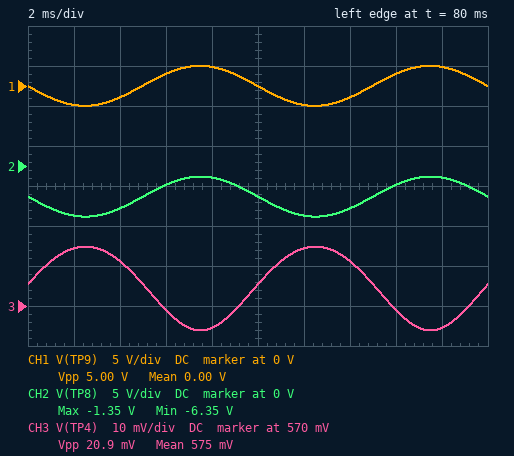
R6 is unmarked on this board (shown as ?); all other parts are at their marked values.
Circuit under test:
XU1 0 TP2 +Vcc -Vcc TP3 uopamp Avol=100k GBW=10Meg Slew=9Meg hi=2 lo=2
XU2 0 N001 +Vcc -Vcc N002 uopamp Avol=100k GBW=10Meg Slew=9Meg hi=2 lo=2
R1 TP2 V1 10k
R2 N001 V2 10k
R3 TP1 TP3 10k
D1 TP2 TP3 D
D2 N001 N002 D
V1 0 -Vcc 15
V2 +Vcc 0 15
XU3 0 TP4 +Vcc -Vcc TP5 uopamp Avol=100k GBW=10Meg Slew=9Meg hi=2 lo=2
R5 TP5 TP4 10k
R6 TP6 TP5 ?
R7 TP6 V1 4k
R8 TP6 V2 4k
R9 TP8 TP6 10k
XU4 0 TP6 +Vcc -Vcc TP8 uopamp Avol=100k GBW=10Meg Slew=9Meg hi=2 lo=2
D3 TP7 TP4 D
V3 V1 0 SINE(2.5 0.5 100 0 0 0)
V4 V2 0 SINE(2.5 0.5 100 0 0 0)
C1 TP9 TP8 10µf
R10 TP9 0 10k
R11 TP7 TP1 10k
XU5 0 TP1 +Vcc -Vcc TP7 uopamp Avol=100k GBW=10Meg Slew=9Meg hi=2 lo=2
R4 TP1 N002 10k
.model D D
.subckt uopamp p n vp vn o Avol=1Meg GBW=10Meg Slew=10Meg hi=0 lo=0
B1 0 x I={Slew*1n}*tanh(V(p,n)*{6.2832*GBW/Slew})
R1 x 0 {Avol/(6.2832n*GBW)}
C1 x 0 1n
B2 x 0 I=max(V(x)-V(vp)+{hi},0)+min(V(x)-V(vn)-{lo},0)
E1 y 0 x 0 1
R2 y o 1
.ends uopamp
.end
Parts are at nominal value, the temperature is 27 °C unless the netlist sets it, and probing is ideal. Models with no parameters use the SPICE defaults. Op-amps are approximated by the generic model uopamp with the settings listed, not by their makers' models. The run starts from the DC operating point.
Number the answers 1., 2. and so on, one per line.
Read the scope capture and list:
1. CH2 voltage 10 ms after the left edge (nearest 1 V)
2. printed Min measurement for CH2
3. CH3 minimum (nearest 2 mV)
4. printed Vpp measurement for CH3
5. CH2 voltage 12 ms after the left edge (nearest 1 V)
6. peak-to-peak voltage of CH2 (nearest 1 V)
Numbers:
1. -4 V
2. -6.35 V
3. 564 mV
4. 20.9 mV
5. -6 V
6. 5 V
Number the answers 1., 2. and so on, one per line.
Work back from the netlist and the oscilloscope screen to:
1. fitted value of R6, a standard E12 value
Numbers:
1. 15 kΩ
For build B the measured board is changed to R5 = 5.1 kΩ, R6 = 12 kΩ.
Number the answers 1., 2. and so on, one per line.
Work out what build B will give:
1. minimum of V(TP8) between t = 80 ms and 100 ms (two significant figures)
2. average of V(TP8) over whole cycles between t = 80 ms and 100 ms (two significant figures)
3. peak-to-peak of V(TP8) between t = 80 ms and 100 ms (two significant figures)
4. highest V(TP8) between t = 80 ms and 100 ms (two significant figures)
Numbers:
1. -4.2 V
2. -1.7 V
3. 5.0 V
4. 840 mV
